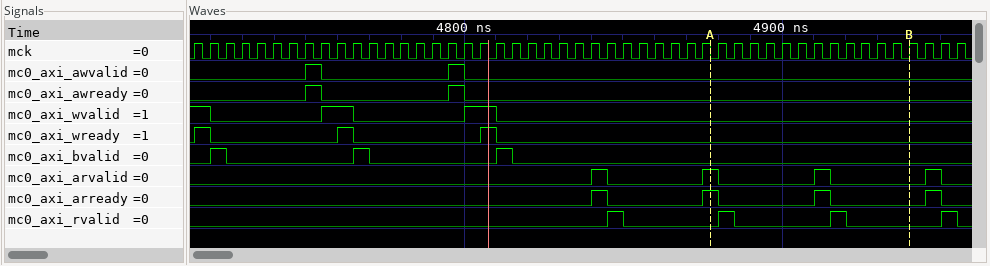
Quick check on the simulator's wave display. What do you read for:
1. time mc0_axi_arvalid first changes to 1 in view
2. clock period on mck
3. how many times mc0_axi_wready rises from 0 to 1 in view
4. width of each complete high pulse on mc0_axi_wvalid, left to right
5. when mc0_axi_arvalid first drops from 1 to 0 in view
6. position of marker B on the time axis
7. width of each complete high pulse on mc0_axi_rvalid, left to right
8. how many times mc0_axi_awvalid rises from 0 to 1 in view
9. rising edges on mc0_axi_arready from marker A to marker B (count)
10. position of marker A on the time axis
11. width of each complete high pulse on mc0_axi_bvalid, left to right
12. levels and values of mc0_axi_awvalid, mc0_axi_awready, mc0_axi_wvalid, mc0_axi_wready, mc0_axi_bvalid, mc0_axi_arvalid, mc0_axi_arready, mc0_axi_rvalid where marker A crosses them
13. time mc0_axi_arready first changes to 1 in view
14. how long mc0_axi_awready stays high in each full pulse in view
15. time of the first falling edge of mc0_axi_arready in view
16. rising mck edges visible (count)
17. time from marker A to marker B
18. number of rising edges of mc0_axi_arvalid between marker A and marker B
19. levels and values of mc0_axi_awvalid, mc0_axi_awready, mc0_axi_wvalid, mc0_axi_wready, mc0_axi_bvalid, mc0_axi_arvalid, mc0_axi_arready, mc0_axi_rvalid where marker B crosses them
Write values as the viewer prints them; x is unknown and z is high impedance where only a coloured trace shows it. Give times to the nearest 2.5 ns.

4840 ns
5 ns
3
10 ns, 10 ns
4845 ns
4940 ns
5 ns, 5 ns, 5 ns, 5 ns
2
1
4877.5 ns
5 ns, 5 ns, 5 ns
mc0_axi_awvalid=0, mc0_axi_awready=0, mc0_axi_wvalid=0, mc0_axi_wready=0, mc0_axi_bvalid=0, mc0_axi_arvalid=1, mc0_axi_arready=1, mc0_axi_rvalid=0
4840 ns
5 ns, 5 ns
4845 ns
49
62.5 ns
1
mc0_axi_awvalid=0, mc0_axi_awready=0, mc0_axi_wvalid=0, mc0_axi_wready=0, mc0_axi_bvalid=0, mc0_axi_arvalid=0, mc0_axi_arready=0, mc0_axi_rvalid=0
